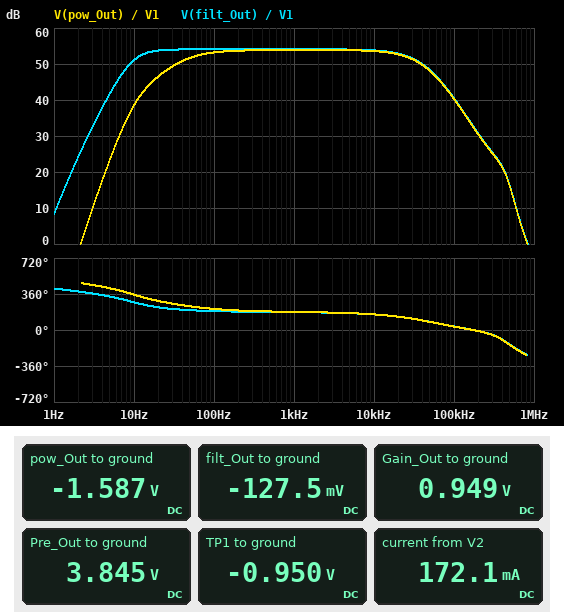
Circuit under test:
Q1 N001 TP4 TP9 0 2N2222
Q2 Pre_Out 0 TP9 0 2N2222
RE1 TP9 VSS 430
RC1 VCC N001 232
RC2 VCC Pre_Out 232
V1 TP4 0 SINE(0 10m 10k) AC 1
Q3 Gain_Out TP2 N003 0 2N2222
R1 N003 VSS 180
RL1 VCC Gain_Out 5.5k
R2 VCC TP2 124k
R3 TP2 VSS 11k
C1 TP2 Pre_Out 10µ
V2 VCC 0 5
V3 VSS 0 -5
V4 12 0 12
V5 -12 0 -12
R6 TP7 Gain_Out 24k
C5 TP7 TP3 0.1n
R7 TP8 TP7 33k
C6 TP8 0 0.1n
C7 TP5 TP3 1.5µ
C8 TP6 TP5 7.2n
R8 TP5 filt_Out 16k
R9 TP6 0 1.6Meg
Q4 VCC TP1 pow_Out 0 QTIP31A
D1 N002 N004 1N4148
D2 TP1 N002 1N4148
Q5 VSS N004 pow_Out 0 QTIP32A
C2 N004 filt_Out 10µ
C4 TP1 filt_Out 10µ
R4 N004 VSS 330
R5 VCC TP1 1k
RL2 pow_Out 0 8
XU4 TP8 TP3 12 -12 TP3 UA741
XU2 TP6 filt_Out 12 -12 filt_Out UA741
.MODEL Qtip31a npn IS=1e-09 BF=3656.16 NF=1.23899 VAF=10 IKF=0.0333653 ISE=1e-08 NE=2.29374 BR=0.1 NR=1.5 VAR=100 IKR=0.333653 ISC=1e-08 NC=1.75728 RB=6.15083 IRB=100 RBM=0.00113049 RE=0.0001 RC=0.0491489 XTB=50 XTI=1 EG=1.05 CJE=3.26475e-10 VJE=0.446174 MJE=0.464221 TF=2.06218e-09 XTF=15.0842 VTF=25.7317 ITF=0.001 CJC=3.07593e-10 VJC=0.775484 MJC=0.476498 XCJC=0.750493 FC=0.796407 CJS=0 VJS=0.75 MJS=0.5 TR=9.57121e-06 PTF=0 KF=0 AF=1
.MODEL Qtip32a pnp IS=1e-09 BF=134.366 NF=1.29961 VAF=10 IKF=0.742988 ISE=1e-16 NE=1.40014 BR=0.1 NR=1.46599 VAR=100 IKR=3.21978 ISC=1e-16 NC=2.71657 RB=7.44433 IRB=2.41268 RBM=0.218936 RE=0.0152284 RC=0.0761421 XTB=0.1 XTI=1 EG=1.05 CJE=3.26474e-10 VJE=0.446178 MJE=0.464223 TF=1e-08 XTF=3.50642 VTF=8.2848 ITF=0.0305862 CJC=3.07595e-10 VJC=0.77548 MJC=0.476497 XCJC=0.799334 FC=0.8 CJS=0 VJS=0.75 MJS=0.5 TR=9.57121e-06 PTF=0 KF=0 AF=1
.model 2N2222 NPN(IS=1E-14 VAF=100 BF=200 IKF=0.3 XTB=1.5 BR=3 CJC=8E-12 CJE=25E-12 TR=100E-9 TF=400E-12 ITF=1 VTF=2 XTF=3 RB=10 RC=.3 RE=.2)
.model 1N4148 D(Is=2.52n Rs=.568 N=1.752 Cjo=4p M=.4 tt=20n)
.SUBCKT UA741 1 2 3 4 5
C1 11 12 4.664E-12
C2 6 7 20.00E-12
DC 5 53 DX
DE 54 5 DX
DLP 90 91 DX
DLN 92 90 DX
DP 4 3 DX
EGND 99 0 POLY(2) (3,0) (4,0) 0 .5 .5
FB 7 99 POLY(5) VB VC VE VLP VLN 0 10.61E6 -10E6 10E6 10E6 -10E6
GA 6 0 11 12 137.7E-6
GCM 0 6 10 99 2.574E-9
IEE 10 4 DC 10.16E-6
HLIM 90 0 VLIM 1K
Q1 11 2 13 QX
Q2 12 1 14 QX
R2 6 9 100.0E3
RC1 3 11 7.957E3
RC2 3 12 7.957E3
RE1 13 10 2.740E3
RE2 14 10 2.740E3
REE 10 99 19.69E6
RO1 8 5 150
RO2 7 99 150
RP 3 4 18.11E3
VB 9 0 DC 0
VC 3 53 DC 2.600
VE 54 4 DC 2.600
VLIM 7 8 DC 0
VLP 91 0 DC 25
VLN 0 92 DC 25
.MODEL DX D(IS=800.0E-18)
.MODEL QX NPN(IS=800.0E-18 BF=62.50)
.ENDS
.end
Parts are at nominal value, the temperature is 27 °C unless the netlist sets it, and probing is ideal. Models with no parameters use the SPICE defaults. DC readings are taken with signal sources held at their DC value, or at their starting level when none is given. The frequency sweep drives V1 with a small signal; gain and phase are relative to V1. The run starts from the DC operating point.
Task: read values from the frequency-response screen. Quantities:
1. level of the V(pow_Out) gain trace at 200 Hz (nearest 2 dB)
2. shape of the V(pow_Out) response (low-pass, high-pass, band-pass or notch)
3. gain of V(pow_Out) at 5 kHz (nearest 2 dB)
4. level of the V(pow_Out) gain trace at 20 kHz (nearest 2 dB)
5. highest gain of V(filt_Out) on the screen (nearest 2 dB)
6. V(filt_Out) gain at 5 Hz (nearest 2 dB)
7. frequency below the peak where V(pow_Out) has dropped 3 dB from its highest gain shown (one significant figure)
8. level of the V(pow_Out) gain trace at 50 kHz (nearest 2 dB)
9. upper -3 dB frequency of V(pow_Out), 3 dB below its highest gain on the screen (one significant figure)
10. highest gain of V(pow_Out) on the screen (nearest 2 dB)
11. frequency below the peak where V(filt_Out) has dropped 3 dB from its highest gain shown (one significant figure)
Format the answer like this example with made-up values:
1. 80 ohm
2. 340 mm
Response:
1. 54 dB
2. band-pass
3. 54 dB
4. 52 dB
5. 54 dB
6. 42 dB
7. 40 Hz
8. 48 dB
9. 30 kHz
10. 54 dB
11. 10 Hz
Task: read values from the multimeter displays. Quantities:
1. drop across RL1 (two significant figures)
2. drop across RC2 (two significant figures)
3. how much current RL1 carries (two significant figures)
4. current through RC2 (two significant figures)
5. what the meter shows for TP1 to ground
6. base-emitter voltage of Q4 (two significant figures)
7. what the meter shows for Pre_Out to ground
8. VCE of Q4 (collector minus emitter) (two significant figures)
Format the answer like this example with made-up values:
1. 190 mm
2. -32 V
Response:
1. 4.1 V
2. 1.2 V
3. 740 µA
4. 5.0 mA
5. -0.950 V
6. 640 mV
7. 3.845 V
8. 6.6 V
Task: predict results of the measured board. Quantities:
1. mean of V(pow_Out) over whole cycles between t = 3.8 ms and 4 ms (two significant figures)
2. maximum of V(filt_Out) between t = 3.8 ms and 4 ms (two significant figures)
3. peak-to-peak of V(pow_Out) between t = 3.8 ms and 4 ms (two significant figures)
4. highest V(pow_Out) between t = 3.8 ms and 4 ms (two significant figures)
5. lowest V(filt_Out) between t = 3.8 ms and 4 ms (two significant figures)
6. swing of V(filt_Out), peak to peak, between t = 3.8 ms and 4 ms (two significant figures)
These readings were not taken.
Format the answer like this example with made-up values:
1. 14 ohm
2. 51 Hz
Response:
1. -1.3 V
2. 3.7 V
3. 7.4 V
4. 2.6 V
5. -3.9 V
6. 7.6 V
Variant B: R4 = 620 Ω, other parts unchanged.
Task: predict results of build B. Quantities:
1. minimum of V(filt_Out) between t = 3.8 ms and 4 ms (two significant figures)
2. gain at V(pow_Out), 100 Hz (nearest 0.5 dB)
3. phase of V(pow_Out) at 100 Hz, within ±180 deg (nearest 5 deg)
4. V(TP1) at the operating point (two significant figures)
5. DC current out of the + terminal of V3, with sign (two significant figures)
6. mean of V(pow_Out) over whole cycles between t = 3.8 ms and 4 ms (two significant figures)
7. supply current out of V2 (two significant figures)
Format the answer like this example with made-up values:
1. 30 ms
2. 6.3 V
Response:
1. -4.9 V
2. 53.5 dB
3. -155 deg
4. 24 mV
5. -260 mA
6. -430 mV
7. 180 mA
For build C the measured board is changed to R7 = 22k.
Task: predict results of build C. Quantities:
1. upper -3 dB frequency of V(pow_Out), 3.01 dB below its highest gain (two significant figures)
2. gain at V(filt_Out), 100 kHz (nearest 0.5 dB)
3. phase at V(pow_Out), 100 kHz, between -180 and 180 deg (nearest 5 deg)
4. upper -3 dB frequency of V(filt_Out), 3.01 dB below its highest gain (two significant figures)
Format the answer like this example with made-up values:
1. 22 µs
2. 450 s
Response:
1. 41 kHz
2. 43.0 dB
3. 45 deg
4. 40 kHz
